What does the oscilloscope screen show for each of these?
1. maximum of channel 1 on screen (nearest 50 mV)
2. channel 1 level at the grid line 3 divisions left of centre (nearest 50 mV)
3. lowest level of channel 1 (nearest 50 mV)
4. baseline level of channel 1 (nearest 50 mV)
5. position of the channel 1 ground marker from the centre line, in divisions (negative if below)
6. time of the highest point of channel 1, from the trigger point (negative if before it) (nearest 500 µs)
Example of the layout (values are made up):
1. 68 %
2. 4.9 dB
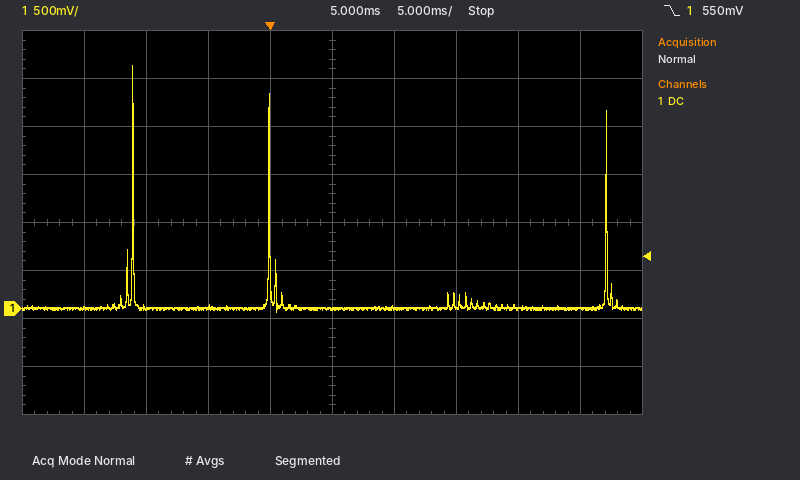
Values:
1. 2.55 V
2. 0 mV
3. -50 mV
4. 0 mV
5. -1.8 div
6. -11.0 ms
